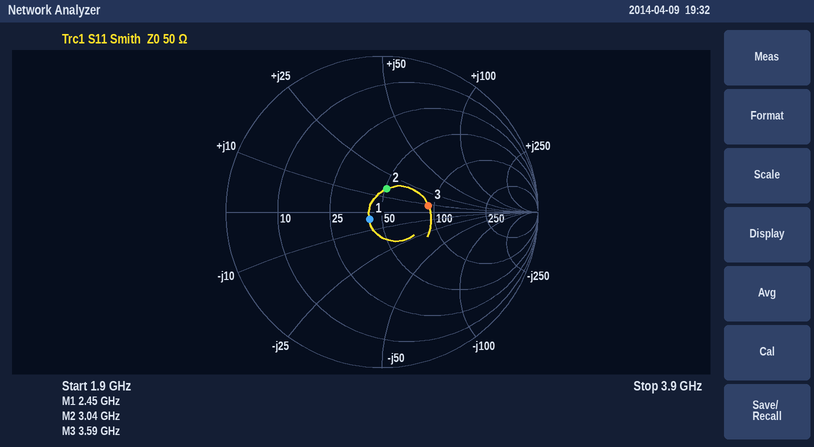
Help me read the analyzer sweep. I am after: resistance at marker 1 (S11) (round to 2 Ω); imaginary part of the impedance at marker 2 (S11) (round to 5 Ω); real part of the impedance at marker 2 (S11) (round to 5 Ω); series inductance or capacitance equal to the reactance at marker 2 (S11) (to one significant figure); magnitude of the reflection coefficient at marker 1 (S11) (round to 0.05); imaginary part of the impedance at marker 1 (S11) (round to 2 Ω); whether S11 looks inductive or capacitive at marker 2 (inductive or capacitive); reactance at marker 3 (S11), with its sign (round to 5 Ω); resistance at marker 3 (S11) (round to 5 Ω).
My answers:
42 Ω
+15 Ω
50 Ω
800 pH
0.10
-4 Ω
inductive
+10 Ω
90 Ω
